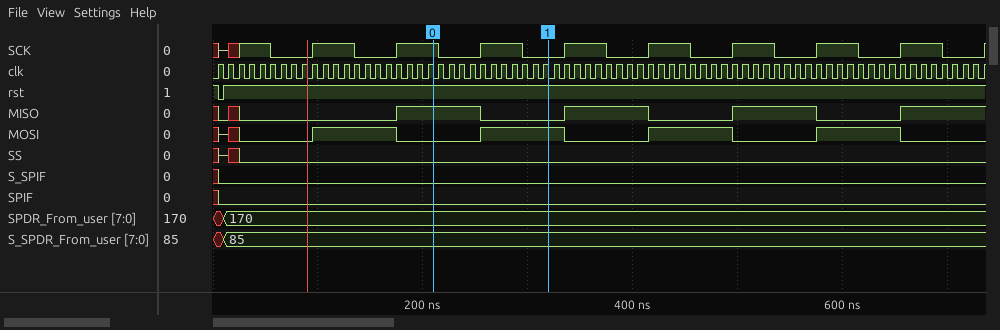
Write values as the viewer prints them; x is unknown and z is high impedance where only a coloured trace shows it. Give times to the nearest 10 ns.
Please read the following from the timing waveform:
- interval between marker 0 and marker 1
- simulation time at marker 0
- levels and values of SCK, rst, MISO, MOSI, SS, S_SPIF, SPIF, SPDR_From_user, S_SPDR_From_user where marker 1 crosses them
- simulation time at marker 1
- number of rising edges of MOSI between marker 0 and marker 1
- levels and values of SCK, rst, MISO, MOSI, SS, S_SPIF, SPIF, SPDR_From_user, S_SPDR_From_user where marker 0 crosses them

110 ns
210 ns
SCK=0, rst=1, MISO=0, MOSI=1, SS=0, S_SPIF=0, SPIF=0, SPDR_From_user=170, S_SPDR_From_user=85
320 ns
1
SCK=1, rst=1, MISO=1, MOSI=0, SS=0, S_SPIF=0, SPIF=0, SPDR_From_user=170, S_SPDR_From_user=85
